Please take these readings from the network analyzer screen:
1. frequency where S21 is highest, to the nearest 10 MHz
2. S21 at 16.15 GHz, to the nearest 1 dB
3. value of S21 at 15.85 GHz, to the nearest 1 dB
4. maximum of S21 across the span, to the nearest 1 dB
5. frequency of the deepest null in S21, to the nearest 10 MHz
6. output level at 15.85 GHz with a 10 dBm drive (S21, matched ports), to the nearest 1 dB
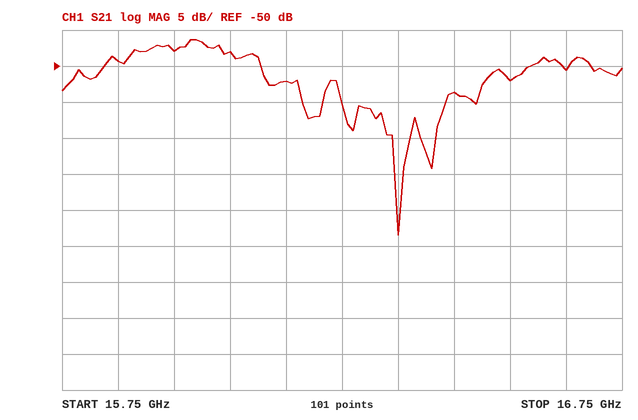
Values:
15.98 GHz
-52 dB
-49 dB
-46 dB
16.35 GHz
-39 dBm
